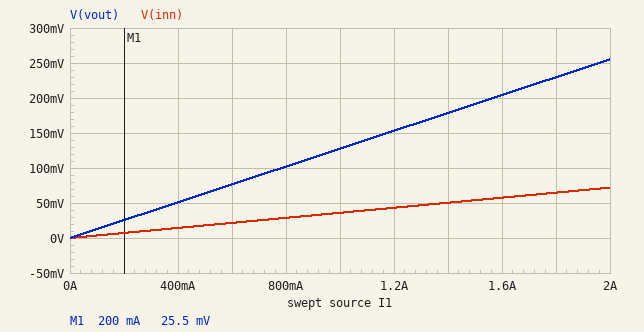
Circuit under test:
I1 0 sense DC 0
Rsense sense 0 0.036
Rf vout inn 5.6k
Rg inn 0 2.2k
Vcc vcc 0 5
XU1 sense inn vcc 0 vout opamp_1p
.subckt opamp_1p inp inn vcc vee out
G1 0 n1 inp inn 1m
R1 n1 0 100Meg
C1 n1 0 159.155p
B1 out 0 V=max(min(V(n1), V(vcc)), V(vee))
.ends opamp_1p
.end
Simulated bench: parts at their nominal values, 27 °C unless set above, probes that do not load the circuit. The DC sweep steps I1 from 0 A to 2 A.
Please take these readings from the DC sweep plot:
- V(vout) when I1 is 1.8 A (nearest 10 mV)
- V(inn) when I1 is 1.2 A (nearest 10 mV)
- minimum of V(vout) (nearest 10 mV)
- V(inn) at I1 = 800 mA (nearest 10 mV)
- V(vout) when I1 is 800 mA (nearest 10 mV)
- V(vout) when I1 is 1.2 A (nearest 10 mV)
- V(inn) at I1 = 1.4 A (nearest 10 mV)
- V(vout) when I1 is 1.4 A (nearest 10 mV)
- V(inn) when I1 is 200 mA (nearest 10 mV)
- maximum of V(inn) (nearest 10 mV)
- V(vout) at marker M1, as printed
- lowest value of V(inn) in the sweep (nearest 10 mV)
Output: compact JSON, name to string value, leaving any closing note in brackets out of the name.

{"V(vout) when I1 is 1.8 A": "230 mV", "V(inn) when I1 is 1.2 A": "40 mV", "minimum of V(vout)": "0 V", "V(inn) at I1 = 800 mA": "30 mV", "V(vout) when I1 is 800 mA": "100 mV", "V(vout) when I1 is 1.2 A": "150 mV", "V(inn) at I1 = 1.4 A": "50 mV", "V(vout) when I1 is 1.4 A": "180 mV", "V(inn) when I1 is 200 mA": "10 mV", "maximum of V(inn)": "70 mV", "V(vout) at marker M1, as printed": "25.5 mV", "lowest value of V(inn) in the sweep": "0 V"}
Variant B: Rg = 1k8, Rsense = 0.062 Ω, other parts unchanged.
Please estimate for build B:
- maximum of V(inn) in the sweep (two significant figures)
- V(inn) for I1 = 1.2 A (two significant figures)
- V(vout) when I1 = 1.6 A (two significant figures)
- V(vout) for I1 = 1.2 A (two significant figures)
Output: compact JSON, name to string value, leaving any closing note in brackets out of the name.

{"maximum of V(inn) in the sweep": "120 mV", "V(inn) for I1 = 1.2 A": "74 mV", "V(vout) when I1 = 1.6 A": "410 mV", "V(vout) for I1 = 1.2 A": "310 mV"}
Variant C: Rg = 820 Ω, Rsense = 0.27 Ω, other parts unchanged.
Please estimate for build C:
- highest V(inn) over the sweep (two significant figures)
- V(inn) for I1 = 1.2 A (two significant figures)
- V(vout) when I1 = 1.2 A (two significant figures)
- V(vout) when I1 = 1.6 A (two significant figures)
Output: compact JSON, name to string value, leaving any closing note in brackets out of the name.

{"highest V(inn) over the sweep": "540 mV", "V(inn) for I1 = 1.2 A": "320 mV", "V(vout) when I1 = 1.2 A": "2.5 V", "V(vout) when I1 = 1.6 A": "3.4 V"}
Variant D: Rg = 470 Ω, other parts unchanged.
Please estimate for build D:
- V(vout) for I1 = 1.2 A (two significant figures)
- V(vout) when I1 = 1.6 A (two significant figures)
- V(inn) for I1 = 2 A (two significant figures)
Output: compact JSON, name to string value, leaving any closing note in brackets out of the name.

{"V(vout) for I1 = 1.2 A": "560 mV", "V(vout) when I1 = 1.6 A": "740 mV", "V(inn) for I1 = 2 A": "72 mV"}
